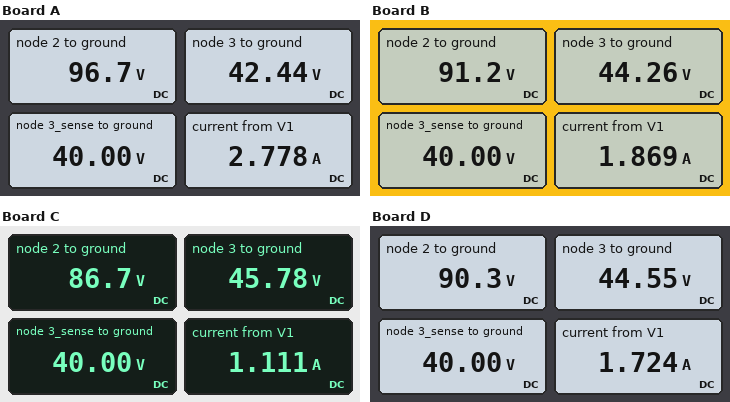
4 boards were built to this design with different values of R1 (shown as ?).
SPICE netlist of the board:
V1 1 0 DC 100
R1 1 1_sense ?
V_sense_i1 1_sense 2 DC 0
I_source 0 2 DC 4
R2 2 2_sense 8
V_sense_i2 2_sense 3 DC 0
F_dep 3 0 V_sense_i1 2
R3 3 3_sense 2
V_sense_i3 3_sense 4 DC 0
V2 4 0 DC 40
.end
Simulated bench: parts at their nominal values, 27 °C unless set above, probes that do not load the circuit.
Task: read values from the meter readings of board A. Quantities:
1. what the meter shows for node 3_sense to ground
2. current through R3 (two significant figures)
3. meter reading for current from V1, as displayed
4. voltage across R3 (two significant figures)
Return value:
40.00 V
1.2 A
2.778 A
2.4 V
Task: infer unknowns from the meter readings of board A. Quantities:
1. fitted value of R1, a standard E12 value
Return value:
1.2 Ω
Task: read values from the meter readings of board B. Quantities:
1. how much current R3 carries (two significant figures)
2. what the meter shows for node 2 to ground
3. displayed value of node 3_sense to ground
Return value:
2.1 A
91.2 V
40.00 V
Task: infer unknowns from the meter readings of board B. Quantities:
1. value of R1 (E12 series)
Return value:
4.7 Ω
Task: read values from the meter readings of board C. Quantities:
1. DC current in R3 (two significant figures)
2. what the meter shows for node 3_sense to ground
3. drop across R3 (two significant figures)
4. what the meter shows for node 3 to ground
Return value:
2.9 A
40.00 V
5.8 V
45.78 V
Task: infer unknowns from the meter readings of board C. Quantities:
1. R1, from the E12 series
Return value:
12 Ω
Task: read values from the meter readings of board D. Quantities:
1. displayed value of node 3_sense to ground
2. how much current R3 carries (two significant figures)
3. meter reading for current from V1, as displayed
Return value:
40.00 V
2.3 A
1.724 A
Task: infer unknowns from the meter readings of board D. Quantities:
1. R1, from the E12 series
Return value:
5.6 Ω
